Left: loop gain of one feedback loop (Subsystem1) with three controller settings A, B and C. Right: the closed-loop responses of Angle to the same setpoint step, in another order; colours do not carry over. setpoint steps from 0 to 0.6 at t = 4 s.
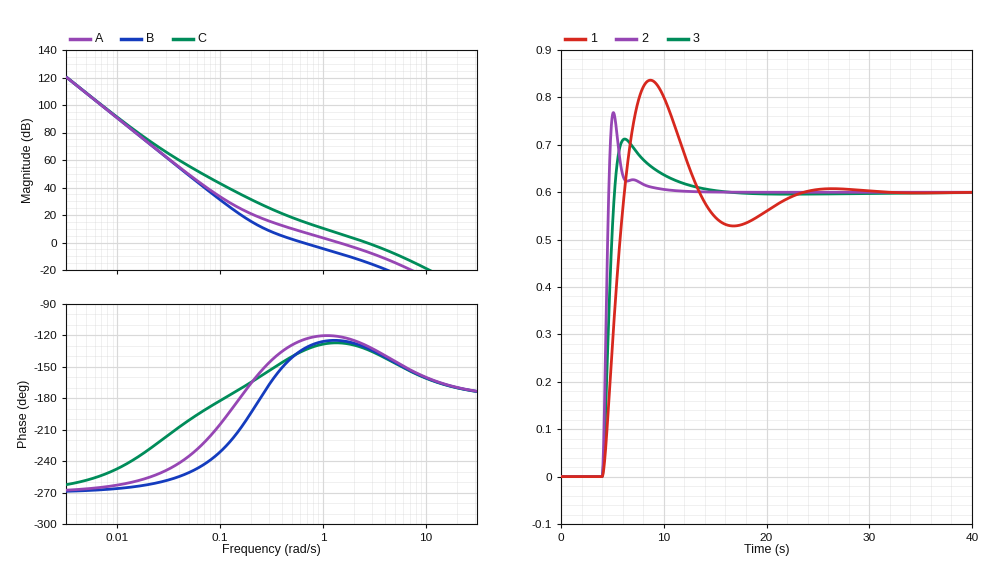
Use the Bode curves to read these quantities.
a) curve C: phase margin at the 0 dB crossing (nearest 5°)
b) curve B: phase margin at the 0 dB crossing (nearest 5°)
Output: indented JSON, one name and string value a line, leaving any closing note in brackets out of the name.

{
  "curve C: phase margin at the 0 dB crossing": "45°",
  "curve B: phase margin at the 0 dB crossing": "45°"
}
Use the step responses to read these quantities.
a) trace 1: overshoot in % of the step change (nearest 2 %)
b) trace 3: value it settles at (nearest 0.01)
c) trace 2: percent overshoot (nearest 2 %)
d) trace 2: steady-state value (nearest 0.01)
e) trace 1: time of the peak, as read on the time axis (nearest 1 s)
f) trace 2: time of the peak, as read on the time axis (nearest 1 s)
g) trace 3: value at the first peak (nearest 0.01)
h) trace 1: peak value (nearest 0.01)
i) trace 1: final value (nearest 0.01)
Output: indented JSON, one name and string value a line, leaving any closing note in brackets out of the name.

{
  "trace 1: overshoot in % of the step change": "40 %",
  "trace 3: value it settles at": "0.60",
  "trace 2: percent overshoot": "28 %",
  "trace 2: steady-state value": "0.60",
  "trace 1: time of the peak, as read on the time axis": "9 s",
  "trace 2: time of the peak, as read on the time axis": "5 s",
  "trace 3: value at the first peak": "0.71",
  "trace 1: peak value": "0.84",
  "trace 1: final value": "0.60"
}
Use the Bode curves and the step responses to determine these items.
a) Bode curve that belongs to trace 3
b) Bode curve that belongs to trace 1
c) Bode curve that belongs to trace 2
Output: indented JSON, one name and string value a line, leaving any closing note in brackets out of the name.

{
  "Bode curve that belongs to trace 3": "A",
  "Bode curve that belongs to trace 1": "B",
  "Bode curve that belongs to trace 2": "C"
}
